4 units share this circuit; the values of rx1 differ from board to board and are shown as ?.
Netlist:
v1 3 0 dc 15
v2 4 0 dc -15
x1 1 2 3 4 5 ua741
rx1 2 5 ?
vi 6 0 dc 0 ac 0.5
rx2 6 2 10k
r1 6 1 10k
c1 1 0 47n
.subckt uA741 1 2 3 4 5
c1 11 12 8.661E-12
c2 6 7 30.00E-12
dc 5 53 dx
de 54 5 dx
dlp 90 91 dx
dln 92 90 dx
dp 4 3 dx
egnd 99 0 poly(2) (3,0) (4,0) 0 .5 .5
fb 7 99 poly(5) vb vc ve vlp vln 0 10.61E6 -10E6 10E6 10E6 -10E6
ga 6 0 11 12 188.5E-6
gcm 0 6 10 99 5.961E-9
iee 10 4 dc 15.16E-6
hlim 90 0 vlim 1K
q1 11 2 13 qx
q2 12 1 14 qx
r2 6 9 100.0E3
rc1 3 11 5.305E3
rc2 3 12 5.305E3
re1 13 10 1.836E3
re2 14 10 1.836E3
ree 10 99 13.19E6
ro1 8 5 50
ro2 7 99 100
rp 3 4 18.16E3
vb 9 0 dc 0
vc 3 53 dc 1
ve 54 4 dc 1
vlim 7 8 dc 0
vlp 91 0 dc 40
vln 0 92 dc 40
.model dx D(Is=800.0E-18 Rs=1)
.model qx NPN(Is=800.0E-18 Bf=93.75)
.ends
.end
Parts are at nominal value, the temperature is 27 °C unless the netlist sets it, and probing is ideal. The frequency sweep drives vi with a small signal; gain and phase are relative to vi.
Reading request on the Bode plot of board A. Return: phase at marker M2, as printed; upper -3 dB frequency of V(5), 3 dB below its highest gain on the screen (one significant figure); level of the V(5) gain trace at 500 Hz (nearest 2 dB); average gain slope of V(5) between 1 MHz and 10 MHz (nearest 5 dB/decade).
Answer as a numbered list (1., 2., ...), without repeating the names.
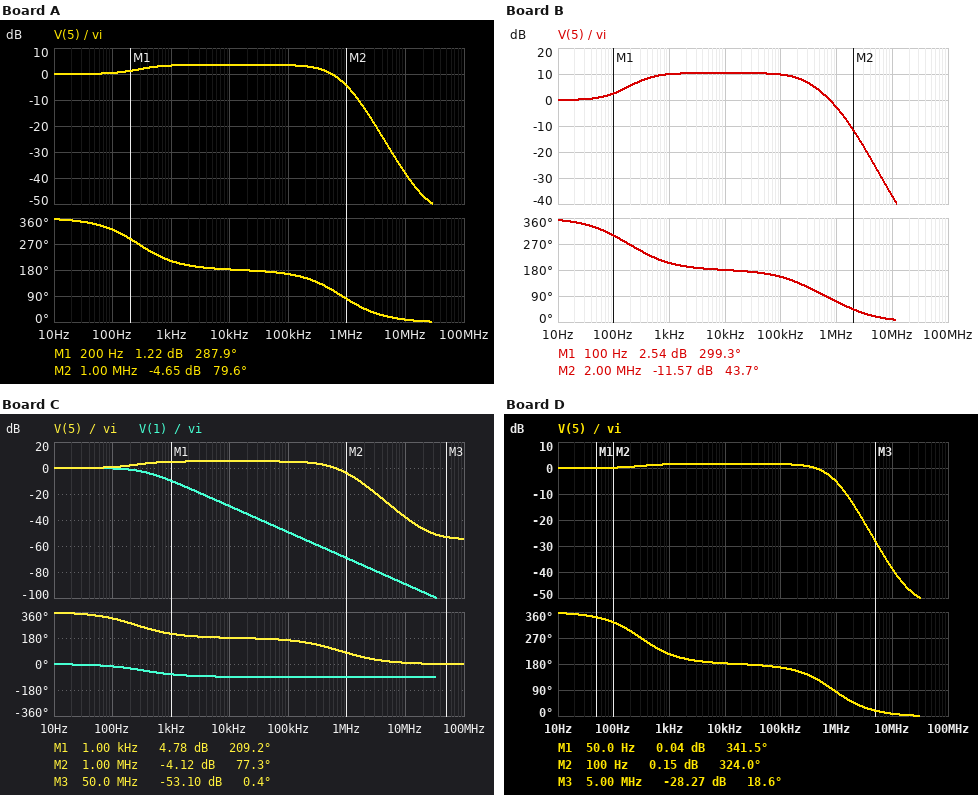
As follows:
1. 79.6 deg
2. 500 kHz
3. 2 dB
4. -35 dB/decade
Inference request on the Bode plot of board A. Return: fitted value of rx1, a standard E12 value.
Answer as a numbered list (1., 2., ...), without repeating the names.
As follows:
1. 15 kΩ
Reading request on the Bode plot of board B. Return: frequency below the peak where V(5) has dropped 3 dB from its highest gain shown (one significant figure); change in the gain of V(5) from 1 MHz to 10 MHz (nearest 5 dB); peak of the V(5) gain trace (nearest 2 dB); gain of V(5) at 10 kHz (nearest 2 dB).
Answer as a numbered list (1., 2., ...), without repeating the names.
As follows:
1. 300 Hz
2. -35 dB
3. 10 dB
4. 10 dB
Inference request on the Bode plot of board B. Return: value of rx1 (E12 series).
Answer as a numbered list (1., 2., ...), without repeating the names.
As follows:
1. 33 kΩ
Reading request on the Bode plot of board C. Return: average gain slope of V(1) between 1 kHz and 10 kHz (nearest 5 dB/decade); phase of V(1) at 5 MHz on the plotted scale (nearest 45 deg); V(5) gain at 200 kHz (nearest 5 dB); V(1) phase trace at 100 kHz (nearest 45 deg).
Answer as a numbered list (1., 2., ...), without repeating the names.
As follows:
1. -20 dB/decade
2. -90 deg
3. 5 dB
4. -90 deg
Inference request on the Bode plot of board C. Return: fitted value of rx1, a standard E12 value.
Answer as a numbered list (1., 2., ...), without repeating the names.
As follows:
1. 18 kΩ
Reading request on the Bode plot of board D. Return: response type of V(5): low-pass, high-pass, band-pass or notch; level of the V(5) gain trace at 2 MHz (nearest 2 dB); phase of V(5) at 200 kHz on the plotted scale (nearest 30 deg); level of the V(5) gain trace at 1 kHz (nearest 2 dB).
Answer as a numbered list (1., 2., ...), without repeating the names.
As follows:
1. low-pass
2. -14 dB
3. 150 deg
4. 2 dB
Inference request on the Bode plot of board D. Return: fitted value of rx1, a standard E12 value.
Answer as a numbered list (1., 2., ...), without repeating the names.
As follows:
1. 12 kΩ
